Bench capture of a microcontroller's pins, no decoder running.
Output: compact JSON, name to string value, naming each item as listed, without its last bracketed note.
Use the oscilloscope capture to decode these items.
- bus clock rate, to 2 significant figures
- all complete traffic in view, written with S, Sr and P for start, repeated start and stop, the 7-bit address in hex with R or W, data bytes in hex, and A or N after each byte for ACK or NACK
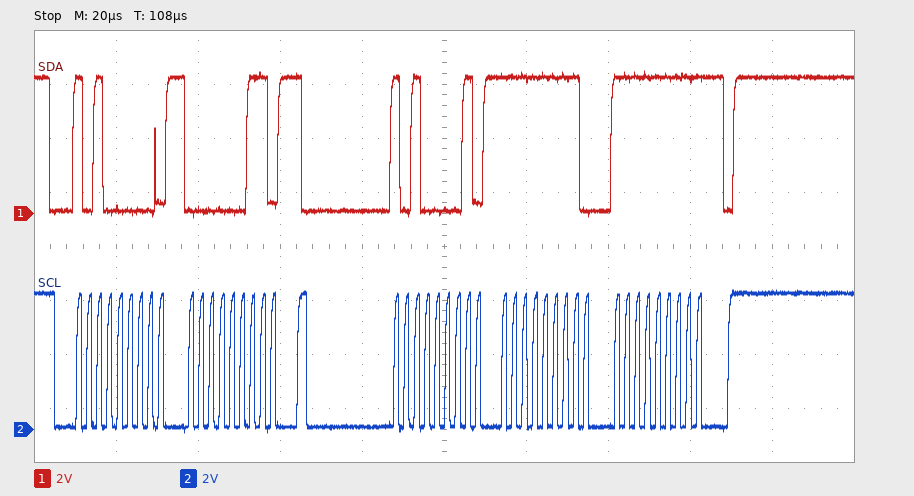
{"bus clock rate, to 2 significant figures": "400 kHz", "all complete traffic in view, written with S, Sr and P for start, repeated start and stop, the 7-bit address in hex with R or W, data bytes in hex, and A or N after each byte for ACK or NACK": "S 50W A 03 A Sr 50R A FF A FF N P"}
